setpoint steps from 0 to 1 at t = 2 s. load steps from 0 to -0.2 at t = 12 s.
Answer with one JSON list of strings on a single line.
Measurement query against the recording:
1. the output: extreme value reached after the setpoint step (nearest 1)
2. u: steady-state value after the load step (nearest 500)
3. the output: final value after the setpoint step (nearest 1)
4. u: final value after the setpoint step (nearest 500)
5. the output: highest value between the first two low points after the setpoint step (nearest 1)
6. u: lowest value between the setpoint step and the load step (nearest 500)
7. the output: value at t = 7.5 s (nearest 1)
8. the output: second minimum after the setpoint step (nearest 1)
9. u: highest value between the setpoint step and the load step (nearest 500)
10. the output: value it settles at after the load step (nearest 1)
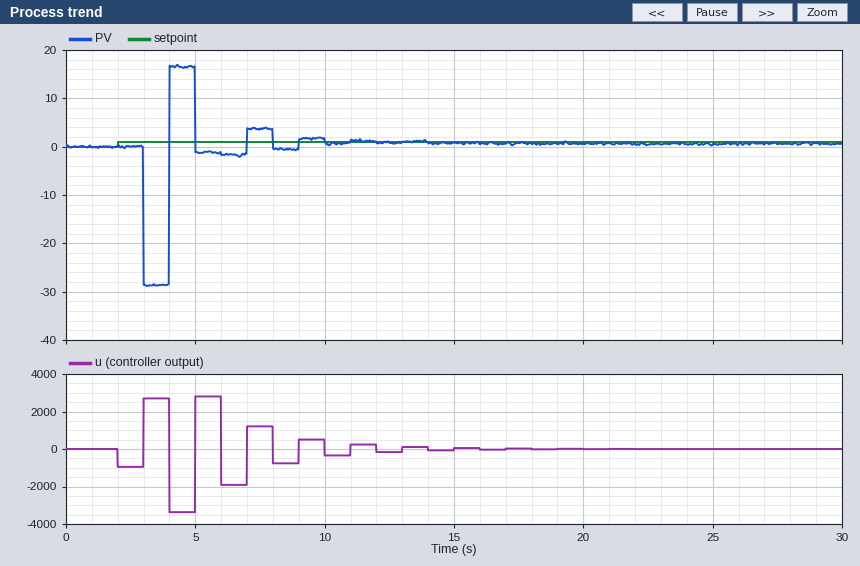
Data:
["-29", "0", "1", "0", "17", "-3500", "4", "-2", "3000", "1"]
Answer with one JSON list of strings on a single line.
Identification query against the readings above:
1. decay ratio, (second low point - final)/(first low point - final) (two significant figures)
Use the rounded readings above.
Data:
["0.10"]
